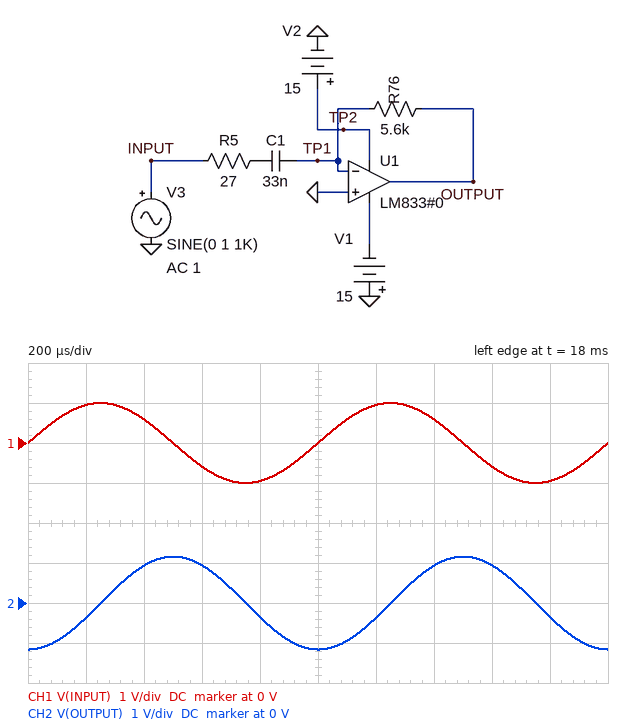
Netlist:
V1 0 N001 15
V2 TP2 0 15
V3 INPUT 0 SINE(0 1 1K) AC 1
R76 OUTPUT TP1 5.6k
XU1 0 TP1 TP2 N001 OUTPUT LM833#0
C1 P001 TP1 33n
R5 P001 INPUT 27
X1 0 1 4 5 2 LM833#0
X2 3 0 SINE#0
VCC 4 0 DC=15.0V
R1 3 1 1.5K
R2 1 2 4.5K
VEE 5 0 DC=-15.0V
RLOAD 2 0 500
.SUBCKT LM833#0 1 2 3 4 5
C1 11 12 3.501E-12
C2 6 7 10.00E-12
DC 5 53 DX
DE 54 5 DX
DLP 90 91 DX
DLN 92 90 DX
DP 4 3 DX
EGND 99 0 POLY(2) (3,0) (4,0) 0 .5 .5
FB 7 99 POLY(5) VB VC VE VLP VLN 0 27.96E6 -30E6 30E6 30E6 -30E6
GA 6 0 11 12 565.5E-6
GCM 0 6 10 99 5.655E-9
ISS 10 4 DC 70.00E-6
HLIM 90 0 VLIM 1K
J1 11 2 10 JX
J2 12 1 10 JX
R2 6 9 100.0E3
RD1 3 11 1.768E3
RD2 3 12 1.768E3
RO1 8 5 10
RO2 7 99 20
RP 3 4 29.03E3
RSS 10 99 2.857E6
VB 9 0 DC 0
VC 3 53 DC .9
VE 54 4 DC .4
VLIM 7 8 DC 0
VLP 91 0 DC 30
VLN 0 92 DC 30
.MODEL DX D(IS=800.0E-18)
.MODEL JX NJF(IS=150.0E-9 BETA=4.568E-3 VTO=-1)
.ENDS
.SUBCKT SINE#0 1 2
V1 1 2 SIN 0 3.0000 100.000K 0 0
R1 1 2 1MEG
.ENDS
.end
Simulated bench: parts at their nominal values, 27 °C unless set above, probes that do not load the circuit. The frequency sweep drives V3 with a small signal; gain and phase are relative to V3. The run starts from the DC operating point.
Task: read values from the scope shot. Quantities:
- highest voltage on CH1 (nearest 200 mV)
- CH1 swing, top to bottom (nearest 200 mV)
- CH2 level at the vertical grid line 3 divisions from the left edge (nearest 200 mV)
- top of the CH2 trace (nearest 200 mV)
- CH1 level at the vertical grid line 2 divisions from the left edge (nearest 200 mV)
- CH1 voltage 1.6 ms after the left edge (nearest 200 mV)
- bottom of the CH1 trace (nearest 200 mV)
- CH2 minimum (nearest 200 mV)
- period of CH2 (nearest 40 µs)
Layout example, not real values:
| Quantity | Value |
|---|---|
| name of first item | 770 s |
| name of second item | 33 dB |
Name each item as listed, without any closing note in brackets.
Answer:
| Quantity | Value |
|---|---|
| highest voltage on CH1 | 1.0 V |
| CH1 swing, top to bottom | 2.0 V |
| CH2 level at the vertical grid line 3 divisions from the left edge | 1.0 V |
| top of the CH2 trace | 1.2 V |
| CH1 level at the vertical grid line 2 divisions from the left edge | 600 mV |
| CH1 voltage 1.6 ms after the left edge | -600 mV |
| bottom of the CH1 trace | -1.0 V |
| CH2 minimum | -1.2 V |
| period of CH2 | 1.00 ms |
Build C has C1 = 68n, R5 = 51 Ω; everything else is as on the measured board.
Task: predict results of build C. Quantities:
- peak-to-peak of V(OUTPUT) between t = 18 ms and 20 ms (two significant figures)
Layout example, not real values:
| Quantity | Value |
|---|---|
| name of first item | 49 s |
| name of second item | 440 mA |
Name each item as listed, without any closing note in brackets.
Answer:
| Quantity | Value |
|---|---|
| peak-to-peak of V(OUTPUT) between t = 18 ms and 20 ms | 4.8 V |
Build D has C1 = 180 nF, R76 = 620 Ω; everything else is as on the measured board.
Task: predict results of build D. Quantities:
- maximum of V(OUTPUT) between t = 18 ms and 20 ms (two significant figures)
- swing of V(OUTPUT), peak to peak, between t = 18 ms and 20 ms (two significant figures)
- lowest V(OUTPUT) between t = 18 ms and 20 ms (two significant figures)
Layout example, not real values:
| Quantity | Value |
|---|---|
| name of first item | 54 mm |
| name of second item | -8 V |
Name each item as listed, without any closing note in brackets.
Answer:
| Quantity | Value |
|---|---|
| maximum of V(OUTPUT) between t = 18 ms and 20 ms | 700 mV |
| swing of V(OUTPUT), peak to peak, between t = 18 ms and 20 ms | 1.4 V |
| lowest V(OUTPUT) between t = 18 ms and 20 ms | -700 mV |
